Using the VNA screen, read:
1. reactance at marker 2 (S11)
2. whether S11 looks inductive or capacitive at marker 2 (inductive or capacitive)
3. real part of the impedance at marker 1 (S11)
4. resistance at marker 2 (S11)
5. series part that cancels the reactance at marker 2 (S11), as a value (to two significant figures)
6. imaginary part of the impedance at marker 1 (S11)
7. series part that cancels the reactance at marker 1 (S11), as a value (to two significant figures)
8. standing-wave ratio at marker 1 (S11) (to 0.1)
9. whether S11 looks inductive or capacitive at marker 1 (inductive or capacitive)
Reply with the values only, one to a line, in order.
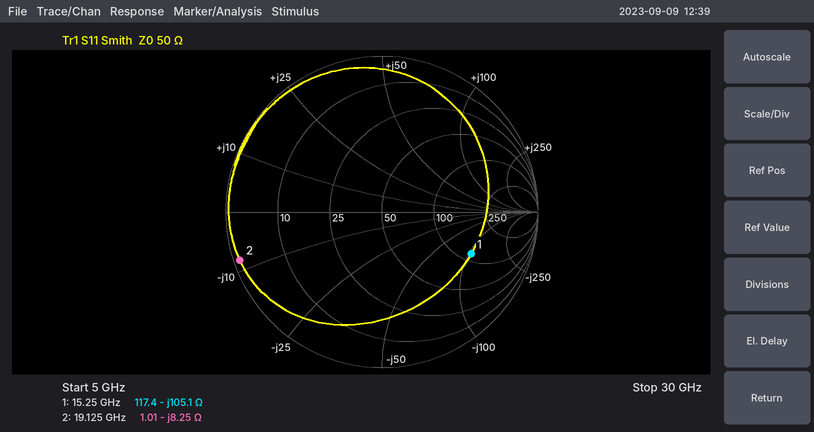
-8.25 Ω
capacitive
117.4 Ω
1.01 Ω
69 pH
-105.1 Ω
1.1 nH
4.4
capacitive
